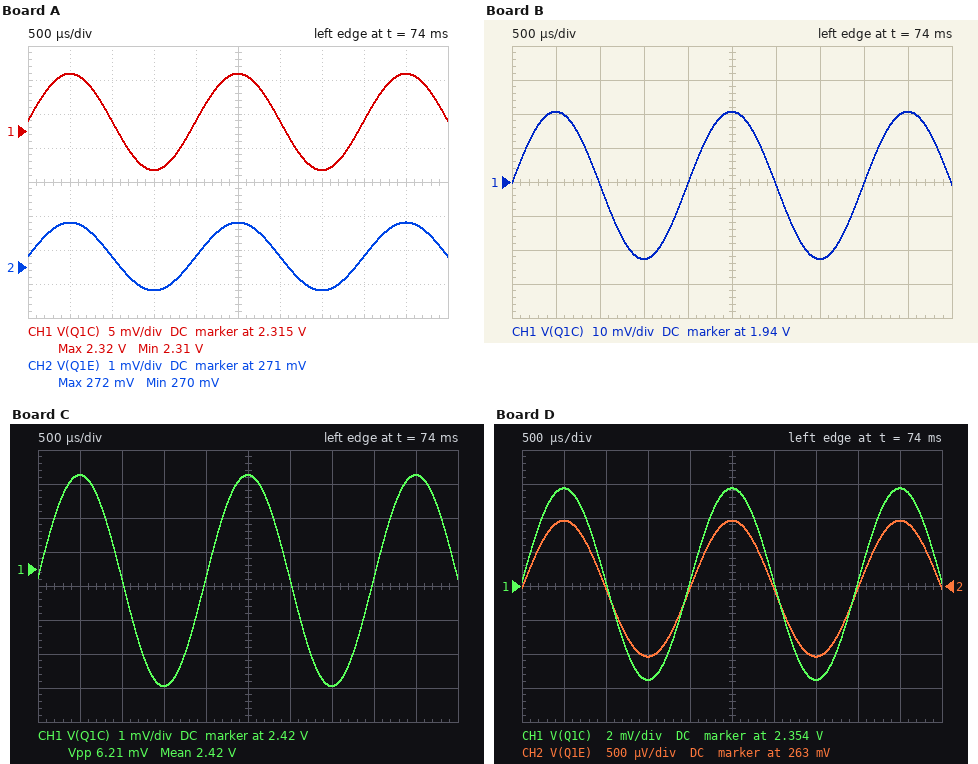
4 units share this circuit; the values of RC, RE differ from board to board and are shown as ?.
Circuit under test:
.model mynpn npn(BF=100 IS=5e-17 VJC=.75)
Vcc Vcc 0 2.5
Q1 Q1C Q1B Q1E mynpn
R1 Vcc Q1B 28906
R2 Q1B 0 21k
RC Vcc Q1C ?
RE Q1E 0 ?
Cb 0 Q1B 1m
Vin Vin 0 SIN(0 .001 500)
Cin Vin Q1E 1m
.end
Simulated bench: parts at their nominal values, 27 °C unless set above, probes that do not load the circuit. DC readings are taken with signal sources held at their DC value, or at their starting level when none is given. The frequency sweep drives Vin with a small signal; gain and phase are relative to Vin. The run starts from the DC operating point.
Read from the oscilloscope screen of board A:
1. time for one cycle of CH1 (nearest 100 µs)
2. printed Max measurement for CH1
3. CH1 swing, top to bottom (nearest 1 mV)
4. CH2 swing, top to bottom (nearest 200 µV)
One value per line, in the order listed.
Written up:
2.0 ms
2.32 V
14 mV
2.0 mV
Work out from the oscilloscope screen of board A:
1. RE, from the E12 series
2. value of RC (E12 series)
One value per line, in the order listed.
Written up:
1.2 kΩ
820 Ω
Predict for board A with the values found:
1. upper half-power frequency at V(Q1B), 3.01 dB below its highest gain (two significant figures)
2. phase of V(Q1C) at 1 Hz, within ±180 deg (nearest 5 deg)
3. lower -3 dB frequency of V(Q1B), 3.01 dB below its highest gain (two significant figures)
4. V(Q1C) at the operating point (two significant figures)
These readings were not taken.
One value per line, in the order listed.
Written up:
1.6 Hz
55 deg
14 mHz
2.3 V
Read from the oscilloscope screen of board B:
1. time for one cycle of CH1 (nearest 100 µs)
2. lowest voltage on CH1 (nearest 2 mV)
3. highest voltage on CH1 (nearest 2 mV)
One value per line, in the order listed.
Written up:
2.0 ms
1.918 V
1.960 V
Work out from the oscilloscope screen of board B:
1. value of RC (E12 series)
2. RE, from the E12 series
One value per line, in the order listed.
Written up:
820 Ω
270 Ω
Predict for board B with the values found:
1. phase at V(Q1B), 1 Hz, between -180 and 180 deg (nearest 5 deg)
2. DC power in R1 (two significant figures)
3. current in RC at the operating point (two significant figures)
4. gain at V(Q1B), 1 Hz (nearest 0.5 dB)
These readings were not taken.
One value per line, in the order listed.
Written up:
-10 deg
81 µW
680 µA
-41.5 dB
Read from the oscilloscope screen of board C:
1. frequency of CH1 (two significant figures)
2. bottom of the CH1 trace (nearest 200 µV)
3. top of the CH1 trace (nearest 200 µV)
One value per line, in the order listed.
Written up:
500 Hz
2.4166 V
2.4228 V
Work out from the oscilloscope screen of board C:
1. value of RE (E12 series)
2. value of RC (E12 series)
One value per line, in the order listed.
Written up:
390 Ω
150 Ω
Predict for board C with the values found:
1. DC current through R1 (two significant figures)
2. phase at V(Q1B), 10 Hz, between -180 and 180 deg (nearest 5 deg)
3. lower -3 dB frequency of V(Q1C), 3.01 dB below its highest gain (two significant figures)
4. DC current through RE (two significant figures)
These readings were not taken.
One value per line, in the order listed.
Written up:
52 µA
-70 deg
3.8 Hz
540 µA
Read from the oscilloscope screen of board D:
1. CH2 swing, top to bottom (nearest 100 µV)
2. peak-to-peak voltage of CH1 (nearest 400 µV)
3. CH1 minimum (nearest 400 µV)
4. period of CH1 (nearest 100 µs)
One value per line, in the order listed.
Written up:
2.0 mV
11.2 mV
2.3484 V
2.0 ms
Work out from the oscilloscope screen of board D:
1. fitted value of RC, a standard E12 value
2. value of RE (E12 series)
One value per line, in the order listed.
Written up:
560 Ω
1 kΩ
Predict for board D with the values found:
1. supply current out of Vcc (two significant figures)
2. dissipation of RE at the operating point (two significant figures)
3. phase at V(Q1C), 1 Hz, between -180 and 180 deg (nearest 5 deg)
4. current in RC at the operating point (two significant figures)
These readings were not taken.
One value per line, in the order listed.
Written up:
310 µA
69 µW
60 deg
260 µA
